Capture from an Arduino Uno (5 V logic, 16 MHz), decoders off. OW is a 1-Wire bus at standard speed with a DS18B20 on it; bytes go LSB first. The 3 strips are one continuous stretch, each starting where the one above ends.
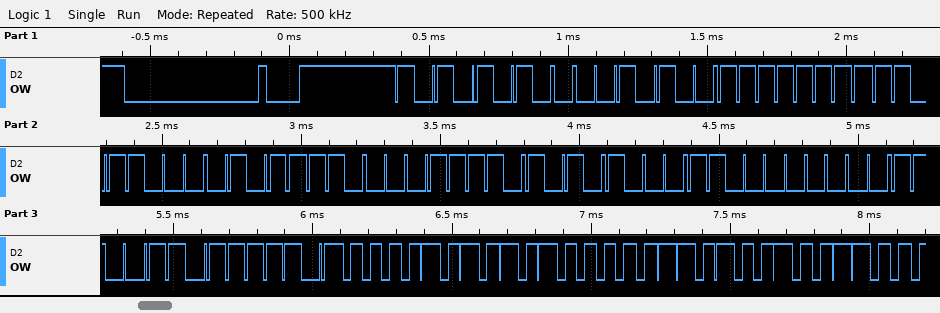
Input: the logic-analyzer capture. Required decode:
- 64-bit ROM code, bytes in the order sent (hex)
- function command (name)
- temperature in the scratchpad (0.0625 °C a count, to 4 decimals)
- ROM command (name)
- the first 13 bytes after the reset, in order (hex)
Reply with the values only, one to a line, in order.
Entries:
28 FF 1B 7A 78 15 03 CC
Read Scratchpad
85.0000 °C
Match ROM
55 28 FF 1B 7A 78 15 03 CC BE 50 05 4B
